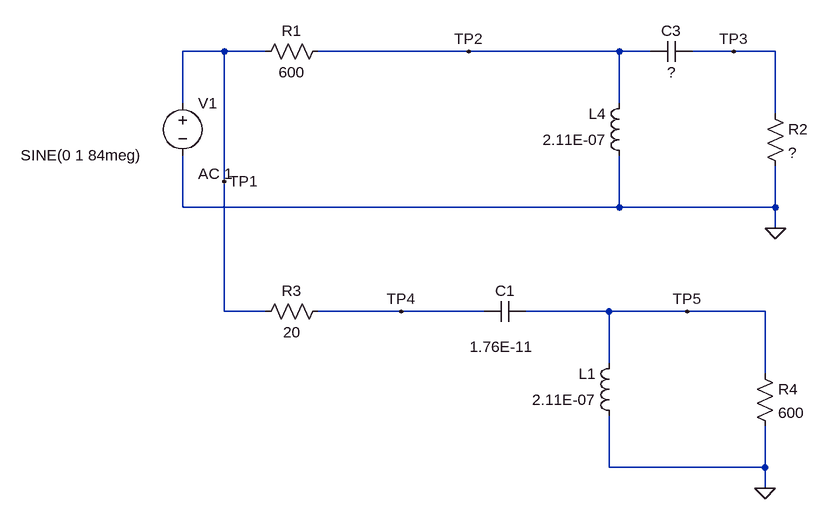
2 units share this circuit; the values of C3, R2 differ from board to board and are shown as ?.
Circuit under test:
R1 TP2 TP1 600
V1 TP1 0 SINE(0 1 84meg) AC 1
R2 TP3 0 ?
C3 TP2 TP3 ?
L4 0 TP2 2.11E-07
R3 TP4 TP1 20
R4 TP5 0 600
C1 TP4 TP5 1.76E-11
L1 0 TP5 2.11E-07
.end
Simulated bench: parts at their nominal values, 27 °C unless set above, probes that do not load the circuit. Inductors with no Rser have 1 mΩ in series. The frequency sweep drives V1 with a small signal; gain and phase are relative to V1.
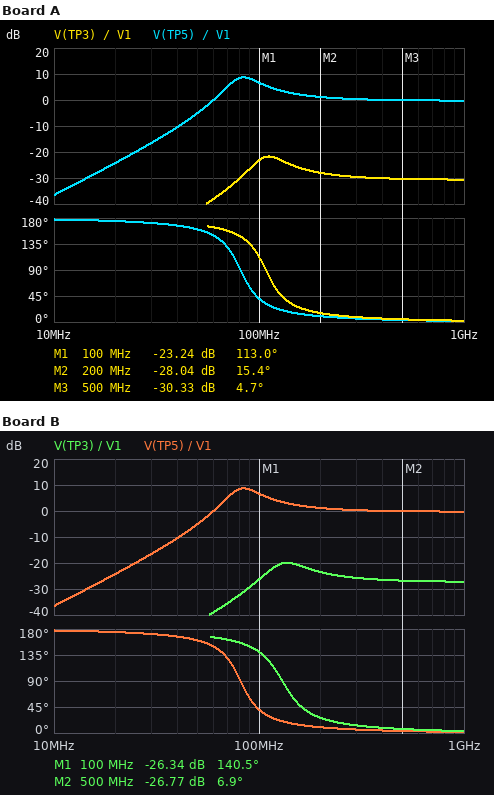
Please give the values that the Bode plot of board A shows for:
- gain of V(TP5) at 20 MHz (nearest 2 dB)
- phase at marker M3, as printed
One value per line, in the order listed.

-24 dB
4.7 deg
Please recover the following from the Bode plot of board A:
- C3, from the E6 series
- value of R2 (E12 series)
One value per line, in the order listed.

10 pF
18 Ω
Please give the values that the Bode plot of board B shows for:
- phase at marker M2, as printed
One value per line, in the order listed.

6.9 deg
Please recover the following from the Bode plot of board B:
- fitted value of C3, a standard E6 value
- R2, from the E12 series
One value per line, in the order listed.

6.8 pF
27 Ω
